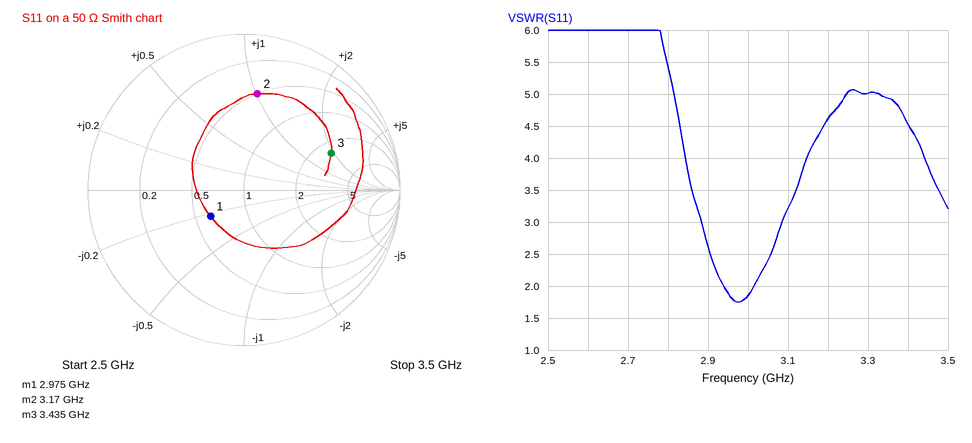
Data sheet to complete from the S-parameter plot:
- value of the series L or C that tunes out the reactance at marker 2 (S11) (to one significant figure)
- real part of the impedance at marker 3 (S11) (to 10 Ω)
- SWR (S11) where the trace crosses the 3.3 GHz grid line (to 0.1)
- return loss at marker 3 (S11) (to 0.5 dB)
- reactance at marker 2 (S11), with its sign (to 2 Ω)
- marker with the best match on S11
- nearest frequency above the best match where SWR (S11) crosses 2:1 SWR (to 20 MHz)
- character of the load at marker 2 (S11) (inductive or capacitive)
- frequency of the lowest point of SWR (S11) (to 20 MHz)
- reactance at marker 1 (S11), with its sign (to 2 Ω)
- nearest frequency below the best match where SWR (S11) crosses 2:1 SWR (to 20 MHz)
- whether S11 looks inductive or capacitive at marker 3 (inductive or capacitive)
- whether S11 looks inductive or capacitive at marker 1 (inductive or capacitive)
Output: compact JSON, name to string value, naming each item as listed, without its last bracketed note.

{"value of the series L or C that tunes out the reactance at marker 2 (S11)": "1.0 pF", "real part of the impedance at marker 3 (S11)": "130 Ω", "SWR (S11) where the trace crosses the 3.3 GHz grid line": "5.0", "return loss at marker 3 (S11)": "4.5 dB", "reactance at marker 2 (S11), with its sign": "+50 Ω", "marker with the best match on S11": "marker 1", "nearest frequency above the best match where SWR (S11) crosses 2:1 SWR": "3.02 GHz", "character of the load at marker 2 (S11)": "inductive", "frequency of the lowest point of SWR (S11)": "2.98 GHz", "reactance at marker 1 (S11), with its sign": "-12 Ω", "nearest frequency below the best match where SWR (S11) crosses 2:1 SWR": "2.94 GHz", "whether S11 looks inductive or capacitive at marker 3": "inductive", "whether S11 looks inductive or capacitive at marker 1": "capacitive"}
